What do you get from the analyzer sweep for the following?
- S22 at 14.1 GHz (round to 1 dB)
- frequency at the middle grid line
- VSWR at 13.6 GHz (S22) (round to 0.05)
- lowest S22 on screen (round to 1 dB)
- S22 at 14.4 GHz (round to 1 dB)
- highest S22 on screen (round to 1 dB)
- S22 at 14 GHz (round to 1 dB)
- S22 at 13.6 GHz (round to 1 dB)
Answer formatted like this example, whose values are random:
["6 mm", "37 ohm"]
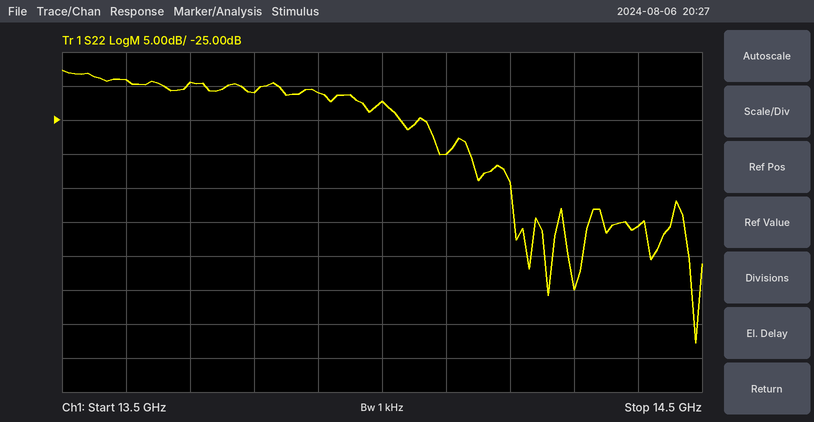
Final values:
["-30 dB", "14 GHz", "1.25", "-58 dB", "-41 dB", "-18 dB", "-22 dB", "-19 dB"]
